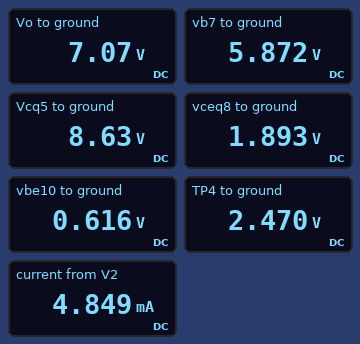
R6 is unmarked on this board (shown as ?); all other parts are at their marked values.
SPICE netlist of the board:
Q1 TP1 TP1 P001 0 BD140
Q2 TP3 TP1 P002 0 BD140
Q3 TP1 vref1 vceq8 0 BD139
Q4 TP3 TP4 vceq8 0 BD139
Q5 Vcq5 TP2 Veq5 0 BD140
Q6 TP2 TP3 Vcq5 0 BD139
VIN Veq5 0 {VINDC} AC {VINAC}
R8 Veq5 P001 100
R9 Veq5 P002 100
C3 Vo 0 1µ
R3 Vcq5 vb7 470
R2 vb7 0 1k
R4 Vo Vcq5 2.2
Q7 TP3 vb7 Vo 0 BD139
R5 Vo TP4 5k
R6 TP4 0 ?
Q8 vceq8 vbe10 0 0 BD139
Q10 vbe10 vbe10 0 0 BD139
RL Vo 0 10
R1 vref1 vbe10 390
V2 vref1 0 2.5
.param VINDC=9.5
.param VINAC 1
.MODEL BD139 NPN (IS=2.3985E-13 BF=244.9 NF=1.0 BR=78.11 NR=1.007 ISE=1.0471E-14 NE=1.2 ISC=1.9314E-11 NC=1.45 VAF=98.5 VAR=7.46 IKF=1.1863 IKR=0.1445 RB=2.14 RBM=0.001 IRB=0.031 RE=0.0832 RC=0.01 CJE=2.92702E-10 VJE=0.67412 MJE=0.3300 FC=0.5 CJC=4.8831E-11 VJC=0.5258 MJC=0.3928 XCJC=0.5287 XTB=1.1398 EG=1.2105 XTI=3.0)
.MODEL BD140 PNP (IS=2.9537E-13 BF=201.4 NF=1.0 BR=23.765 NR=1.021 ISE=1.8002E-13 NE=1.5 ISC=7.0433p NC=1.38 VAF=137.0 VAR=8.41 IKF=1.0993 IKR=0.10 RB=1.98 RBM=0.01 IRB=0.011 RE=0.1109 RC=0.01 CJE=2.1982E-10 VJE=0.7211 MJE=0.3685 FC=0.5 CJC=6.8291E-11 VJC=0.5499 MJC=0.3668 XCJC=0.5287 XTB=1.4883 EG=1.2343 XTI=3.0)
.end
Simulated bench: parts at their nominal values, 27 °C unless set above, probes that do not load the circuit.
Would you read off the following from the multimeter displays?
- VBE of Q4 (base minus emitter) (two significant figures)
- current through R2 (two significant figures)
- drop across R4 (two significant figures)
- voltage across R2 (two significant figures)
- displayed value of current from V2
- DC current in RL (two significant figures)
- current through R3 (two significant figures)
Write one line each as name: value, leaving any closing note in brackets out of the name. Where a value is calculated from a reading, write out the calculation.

VBE of Q4 (base minus emitter): 2.47 V - 1.893 V = 580 mV
current through R2: (5.872 V) / 1 kΩ = 5.9 mA
drop across R4: 8.63 V - 7.07 V = 1.6 V
voltage across R2: 5.872 V = 5.9 V
displayed value of current from V2: 4.849 mA
DC current in RL: (7.07 V) / 10 Ω = 710 mA
current through R3: (8.63 V - 5.872 V) / 470 Ω = 5.9 mA
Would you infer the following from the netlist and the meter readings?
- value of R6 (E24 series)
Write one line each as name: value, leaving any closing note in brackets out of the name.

value of R6: 2.7 kΩ
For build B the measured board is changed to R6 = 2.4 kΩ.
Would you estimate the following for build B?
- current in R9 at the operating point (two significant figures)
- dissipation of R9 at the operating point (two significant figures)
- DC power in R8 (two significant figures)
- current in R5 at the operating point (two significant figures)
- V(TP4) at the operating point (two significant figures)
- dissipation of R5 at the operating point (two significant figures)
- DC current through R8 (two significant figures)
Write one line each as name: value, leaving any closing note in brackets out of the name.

current in R9 at the operating point: 2.3 mA
dissipation of R9 at the operating point: 540 µW
DC power in R8: 840 µW
current in R5 at the operating point: 960 µA
V(TP4) at the operating point: 2.3 V
dissipation of R5 at the operating point: 4.6 mW
DC current through R8: 2.9 mA
